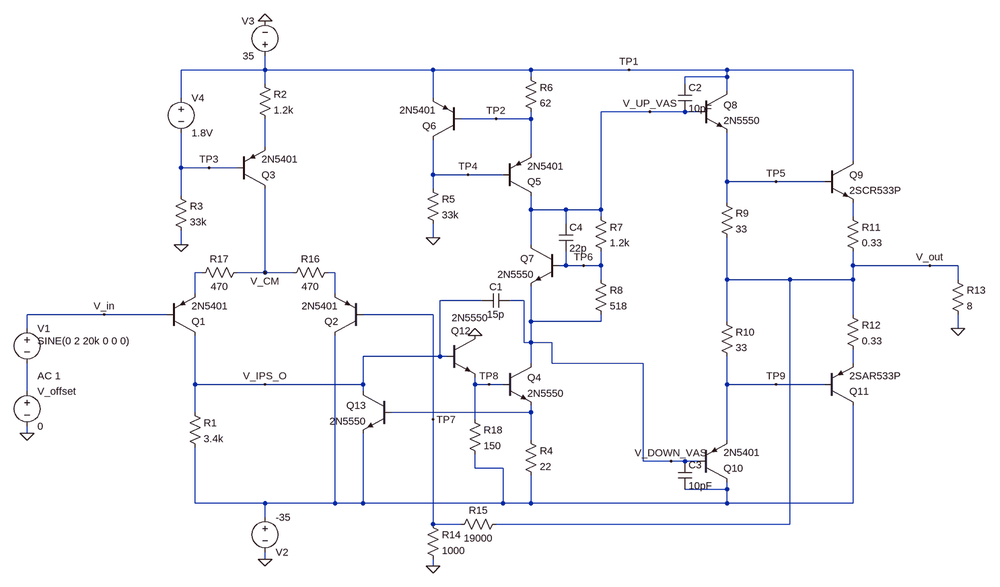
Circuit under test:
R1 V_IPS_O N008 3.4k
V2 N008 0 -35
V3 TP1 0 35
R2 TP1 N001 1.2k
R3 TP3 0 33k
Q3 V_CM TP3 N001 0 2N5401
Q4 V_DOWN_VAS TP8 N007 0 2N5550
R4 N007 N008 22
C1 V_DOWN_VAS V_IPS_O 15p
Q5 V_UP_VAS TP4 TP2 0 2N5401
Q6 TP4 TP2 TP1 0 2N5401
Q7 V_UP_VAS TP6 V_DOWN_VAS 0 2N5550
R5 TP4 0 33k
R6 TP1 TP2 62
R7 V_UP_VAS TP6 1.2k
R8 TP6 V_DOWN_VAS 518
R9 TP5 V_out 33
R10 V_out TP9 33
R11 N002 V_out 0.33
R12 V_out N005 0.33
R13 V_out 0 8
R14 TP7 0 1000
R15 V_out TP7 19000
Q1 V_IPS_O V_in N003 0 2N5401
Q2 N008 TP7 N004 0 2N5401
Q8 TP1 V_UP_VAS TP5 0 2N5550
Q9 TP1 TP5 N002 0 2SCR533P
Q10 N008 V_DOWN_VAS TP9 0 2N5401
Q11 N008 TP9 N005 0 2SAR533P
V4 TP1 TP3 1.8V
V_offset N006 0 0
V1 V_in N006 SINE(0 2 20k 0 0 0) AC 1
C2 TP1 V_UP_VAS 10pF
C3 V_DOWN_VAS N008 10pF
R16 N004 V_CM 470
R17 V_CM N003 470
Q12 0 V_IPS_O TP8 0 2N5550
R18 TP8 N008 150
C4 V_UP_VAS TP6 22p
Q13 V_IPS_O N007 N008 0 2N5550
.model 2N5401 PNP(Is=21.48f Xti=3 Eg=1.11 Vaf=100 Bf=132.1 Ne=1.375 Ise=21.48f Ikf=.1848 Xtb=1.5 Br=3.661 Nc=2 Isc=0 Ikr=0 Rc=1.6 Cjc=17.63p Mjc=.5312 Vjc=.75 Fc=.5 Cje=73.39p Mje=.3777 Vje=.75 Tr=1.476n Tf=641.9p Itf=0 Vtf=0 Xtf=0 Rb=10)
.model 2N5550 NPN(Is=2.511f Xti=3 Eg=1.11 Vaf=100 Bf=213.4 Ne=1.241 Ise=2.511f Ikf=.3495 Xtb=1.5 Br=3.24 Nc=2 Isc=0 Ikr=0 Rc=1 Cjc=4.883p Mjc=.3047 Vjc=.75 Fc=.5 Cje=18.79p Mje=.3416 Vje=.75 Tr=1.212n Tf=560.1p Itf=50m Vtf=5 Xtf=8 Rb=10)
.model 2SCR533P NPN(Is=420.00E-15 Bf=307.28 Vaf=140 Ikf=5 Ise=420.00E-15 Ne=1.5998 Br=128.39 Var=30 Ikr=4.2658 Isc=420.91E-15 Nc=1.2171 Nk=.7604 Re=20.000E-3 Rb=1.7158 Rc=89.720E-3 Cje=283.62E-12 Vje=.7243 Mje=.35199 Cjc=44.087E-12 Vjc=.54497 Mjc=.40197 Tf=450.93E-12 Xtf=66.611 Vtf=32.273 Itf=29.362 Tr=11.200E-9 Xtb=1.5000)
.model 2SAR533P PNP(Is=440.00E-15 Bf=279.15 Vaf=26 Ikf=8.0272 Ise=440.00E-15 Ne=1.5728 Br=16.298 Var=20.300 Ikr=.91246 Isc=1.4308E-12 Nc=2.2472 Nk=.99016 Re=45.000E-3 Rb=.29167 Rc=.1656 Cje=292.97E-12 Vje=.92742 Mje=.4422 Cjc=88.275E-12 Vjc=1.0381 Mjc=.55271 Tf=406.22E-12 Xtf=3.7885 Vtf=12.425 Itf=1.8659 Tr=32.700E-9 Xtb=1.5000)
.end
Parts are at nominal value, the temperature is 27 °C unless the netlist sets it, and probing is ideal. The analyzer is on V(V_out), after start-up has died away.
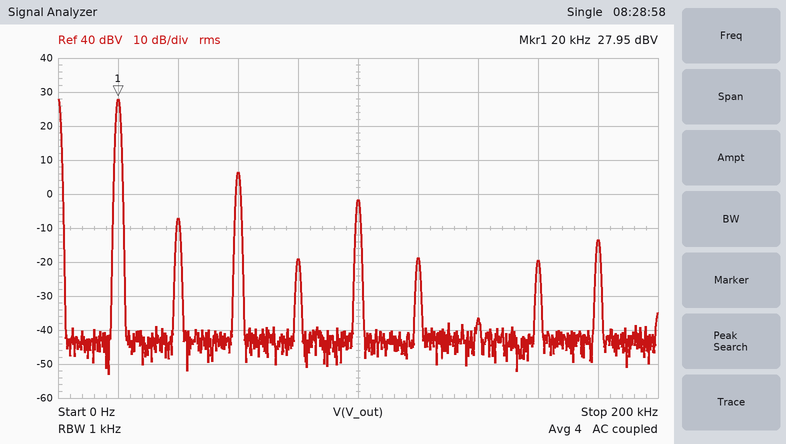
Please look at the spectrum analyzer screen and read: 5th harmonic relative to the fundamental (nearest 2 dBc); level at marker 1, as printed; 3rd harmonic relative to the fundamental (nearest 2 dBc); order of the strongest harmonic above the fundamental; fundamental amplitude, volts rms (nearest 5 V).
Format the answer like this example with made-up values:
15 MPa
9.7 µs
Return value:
-30 dBc
27.95 dBV
-22 dBc
3
25 V
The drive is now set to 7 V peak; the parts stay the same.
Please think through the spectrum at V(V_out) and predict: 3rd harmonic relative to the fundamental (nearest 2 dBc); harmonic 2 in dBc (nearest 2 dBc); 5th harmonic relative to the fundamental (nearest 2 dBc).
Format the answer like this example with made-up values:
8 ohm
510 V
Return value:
-10 dBc
-42 dBc
-16 dBc
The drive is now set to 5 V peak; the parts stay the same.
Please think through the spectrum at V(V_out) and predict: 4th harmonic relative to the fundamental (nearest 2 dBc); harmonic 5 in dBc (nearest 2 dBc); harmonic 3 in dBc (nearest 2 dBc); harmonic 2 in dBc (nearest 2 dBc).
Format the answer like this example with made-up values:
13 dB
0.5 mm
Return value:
-42 dBc
-18 dBc
-10 dBc
-40 dBc
